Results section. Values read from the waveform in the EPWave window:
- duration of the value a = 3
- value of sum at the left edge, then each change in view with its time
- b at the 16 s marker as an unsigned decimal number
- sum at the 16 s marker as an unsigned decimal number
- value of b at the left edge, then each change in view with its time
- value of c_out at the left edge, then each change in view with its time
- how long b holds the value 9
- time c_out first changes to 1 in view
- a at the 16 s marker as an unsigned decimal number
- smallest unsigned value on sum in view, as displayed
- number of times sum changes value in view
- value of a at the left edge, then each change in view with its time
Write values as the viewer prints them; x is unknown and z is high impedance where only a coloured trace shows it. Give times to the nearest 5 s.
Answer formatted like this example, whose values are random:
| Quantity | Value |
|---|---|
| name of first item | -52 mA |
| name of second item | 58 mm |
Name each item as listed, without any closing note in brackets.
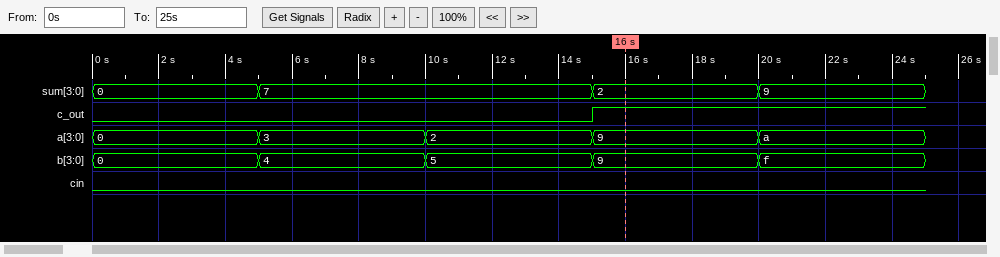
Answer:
| Quantity | Value |
|---|---|
| duration of the value a = 3 | 5 s |
| value of sum at the left edge, then each change in view with its time | 0, 7 at 5 s, 2 at 15 s, 9 at 20 s |
| b at the 16 s marker as an unsigned decimal number | 9 |
| sum at the 16 s marker as an unsigned decimal number | 2 |
| value of b at the left edge, then each change in view with its time | 0, 4 at 5 s, 5 at 10 s, 9 at 15 s, f at 20 s |
| value of c_out at the left edge, then each change in view with its time | 0, 1 at 15 s |
| how long b holds the value 9 | 5 s |
| time c_out first changes to 1 in view | 15 s |
| a at the 16 s marker as an unsigned decimal number | 9 |
| smallest unsigned value on sum in view, as displayed | 0 |
| number of times sum changes value in view | 3 |
| value of a at the left edge, then each change in view with its time | 0, 3 at 5 s, 2 at 10 s, 9 at 15 s, a at 20 s |
